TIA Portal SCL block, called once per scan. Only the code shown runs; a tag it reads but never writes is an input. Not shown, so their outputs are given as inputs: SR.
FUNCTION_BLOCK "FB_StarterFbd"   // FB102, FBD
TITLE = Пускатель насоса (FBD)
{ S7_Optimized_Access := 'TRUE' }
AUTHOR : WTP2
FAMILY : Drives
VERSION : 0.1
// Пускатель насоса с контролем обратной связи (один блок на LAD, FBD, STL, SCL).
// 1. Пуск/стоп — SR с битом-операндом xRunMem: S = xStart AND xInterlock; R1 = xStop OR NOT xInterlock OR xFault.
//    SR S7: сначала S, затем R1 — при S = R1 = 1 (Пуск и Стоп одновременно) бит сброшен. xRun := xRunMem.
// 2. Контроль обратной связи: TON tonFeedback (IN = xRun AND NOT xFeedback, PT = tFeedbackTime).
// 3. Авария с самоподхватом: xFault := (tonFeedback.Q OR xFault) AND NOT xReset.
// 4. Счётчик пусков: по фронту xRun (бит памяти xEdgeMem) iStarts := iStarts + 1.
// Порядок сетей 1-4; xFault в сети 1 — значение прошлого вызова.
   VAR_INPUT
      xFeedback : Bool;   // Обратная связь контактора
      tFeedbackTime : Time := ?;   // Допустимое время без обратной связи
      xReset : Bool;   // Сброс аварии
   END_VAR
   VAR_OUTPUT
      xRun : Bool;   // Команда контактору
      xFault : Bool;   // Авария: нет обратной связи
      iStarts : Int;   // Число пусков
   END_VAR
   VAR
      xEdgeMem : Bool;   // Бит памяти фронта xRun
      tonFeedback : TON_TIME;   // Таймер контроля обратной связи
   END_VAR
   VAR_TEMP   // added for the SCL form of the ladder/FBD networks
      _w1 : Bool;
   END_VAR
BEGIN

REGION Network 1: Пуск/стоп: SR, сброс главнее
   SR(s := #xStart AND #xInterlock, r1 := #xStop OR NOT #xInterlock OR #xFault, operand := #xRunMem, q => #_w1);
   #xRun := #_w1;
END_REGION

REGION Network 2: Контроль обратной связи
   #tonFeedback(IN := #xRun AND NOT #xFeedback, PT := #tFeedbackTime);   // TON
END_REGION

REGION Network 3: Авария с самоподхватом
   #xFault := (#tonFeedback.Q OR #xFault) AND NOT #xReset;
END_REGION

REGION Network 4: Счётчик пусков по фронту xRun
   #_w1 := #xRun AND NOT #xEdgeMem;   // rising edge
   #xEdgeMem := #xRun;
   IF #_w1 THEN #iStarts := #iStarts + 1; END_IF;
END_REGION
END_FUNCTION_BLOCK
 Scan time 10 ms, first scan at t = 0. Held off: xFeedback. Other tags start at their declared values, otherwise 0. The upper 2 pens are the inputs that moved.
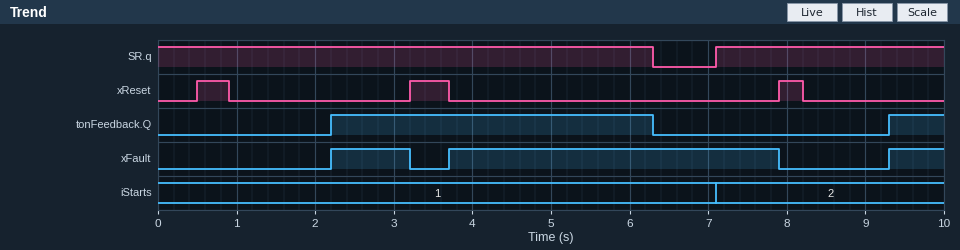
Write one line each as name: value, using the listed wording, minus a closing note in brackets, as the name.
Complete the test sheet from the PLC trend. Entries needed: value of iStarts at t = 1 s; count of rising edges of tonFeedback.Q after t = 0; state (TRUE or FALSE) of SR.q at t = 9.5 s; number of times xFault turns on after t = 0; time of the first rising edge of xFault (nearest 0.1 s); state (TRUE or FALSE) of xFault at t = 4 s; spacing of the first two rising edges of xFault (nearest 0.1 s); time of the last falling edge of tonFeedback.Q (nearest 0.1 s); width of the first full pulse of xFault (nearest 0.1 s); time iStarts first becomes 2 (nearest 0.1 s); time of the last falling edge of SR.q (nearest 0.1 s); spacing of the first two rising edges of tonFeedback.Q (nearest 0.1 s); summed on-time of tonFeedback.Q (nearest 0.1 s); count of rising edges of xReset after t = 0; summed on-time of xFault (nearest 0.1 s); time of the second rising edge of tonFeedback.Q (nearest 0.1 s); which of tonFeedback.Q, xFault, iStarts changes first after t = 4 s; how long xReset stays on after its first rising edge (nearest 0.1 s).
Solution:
value of iStarts at t = 1 s: 1
count of rising edges of tonFeedback.Q after t = 0: 2
state (TRUE or FALSE) of SR.q at t = 9.5 s: TRUE
number of times xFault turns on after t = 0: 3
time of the first rising edge of xFault: 2.2 s
state (TRUE or FALSE) of xFault at t = 4 s: TRUE
spacing of the first two rising edges of xFault: 1.5 s
time of the last falling edge of tonFeedback.Q: 6.3 s
width of the first full pulse of xFault: 1.0 s
time iStarts first becomes 2: 7.1 s
time of the last falling edge of SR.q: 6.3 s
spacing of the first two rising edges of tonFeedback.Q: 7.1 s
summed on-time of tonFeedback.Q: 4.8 s
count of rising edges of xReset after t = 0: 3
summed on-time of xFault: 5.9 s
time of the second rising edge of tonFeedback.Q: 9.3 s
which of tonFeedback.Q, xFault, iStarts changes first after t = 4 s: tonFeedback.Q
how long xReset stays on after its first rising edge: 0.4 s
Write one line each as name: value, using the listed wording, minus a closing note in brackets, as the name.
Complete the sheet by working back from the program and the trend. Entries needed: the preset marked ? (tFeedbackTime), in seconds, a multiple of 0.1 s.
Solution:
the preset marked ? (tFeedbackTime), in seconds, a multiple of 0.1 s: 2.2 s
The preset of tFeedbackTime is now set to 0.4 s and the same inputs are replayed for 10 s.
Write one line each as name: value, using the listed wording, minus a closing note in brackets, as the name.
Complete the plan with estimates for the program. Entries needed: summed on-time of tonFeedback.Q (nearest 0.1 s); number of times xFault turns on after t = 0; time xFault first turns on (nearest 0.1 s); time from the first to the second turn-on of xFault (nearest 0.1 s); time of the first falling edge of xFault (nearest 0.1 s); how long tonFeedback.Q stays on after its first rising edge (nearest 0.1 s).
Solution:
summed on-time of tonFeedback.Q: 8.4 s
number of times xFault turns on after t = 0: 4
time xFault first turns on: 0.4 s
time from the first to the second turn-on of xFault: 0.5 s
time of the first falling edge of xFault: 0.5 s
how long tonFeedback.Q stays on after its first rising edge: 5.9 s
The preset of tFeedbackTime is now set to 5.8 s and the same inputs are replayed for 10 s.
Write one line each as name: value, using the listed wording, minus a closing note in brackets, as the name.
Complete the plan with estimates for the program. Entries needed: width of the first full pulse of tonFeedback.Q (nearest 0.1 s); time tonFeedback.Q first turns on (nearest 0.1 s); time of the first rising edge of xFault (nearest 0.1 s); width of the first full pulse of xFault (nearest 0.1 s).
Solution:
width of the first full pulse of tonFeedback.Q: 0.5 s
time tonFeedback.Q first turns on: 5.8 s
time of the first rising edge of xFault: 5.8 s
width of the first full pulse of xFault: 2.1 s
